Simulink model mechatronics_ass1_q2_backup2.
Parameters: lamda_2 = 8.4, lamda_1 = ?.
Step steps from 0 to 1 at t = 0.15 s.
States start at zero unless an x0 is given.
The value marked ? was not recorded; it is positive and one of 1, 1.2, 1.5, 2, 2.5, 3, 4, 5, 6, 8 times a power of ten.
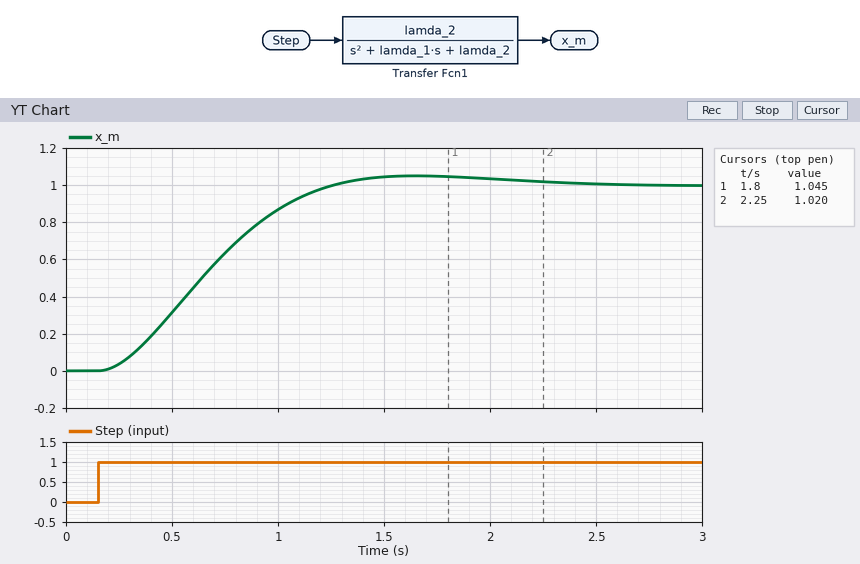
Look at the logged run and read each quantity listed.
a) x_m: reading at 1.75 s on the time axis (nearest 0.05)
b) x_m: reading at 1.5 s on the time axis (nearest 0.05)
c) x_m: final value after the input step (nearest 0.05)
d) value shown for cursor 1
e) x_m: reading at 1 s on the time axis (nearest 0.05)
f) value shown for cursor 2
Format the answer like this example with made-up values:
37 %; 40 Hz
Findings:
1.05; 1.05; 1.00; 1.045; 0.85; 1.020
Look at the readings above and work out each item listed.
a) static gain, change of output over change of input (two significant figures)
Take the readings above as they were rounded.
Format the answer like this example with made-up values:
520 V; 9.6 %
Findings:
1.0
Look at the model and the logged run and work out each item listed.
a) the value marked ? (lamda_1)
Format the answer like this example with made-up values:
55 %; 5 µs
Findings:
4
